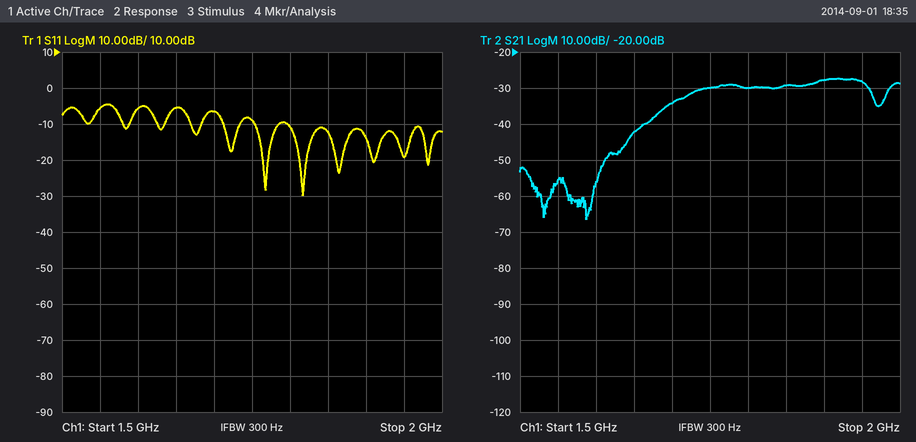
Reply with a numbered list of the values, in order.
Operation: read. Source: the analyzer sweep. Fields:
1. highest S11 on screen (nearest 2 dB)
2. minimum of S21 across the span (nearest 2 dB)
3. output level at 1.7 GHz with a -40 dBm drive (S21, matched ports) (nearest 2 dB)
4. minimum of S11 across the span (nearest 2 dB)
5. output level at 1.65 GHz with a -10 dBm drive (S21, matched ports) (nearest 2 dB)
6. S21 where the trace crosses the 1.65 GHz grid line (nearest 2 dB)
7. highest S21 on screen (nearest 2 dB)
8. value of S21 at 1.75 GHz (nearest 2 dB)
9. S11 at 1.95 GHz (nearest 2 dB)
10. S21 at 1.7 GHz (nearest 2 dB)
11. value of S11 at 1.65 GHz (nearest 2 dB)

1. -4 dB
2. -66 dB
3. -74 dBm
4. -30 dB
5. -52 dBm
6. -42 dB
7. -28 dB
8. -30 dB
9. -20 dB
10. -34 dB
11. -6 dB
